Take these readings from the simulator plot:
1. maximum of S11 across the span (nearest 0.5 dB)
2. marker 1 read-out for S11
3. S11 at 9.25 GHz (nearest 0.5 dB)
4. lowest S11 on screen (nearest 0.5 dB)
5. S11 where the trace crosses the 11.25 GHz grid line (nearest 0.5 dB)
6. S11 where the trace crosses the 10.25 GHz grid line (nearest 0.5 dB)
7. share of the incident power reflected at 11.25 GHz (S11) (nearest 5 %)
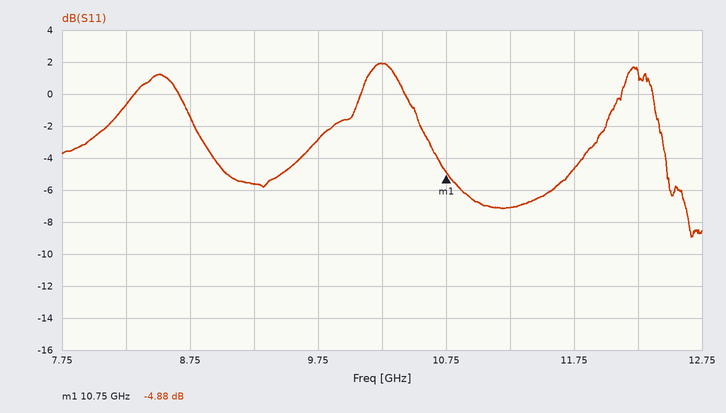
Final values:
2.0 dB
-4.88 dB
-5.5 dB
-9.0 dB
-7.0 dB
2.0 dB
20 %
